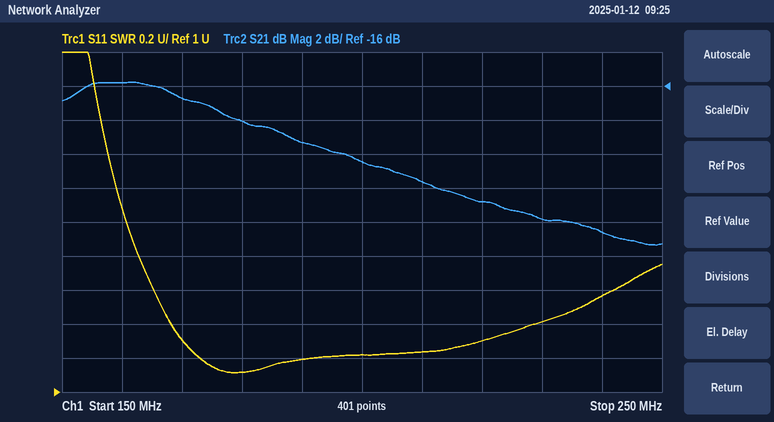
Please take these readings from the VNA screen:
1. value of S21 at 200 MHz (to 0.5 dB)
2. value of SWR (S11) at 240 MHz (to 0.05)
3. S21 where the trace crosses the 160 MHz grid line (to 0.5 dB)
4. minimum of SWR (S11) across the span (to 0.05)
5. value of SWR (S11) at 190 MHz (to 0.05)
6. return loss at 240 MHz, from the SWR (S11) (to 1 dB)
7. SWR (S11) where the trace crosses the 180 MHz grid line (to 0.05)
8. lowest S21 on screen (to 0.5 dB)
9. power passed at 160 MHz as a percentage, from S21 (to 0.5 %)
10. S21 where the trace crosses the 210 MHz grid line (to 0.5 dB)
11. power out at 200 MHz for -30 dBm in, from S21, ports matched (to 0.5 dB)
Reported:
-20.5 dB
1.55
-16.0 dB
1.10
1.20
13 dB
1.10
-25.5 dB
2.5 %
-21.5 dB
-50.5 dBm
